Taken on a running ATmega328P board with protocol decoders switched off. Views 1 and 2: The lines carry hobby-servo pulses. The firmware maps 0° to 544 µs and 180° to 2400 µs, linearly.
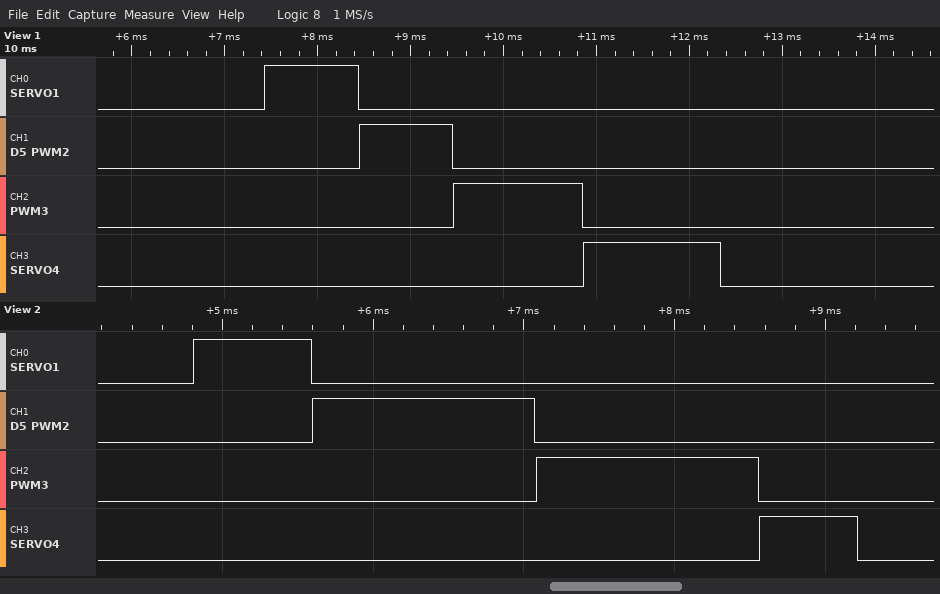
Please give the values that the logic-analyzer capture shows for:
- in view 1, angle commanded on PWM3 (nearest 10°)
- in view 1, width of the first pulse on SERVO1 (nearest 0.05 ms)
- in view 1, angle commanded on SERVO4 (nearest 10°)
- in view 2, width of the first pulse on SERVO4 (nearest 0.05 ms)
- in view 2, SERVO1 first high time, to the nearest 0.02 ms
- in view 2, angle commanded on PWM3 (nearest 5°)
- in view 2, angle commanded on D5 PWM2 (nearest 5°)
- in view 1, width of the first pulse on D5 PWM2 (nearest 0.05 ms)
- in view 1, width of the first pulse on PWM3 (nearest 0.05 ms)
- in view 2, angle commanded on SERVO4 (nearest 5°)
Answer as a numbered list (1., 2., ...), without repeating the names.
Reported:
1. 80°
2. 1.00 ms
3. 90°
4. 0.65 ms
5. 0.78 ms
6. 90°
7. 90°
8. 1.00 ms
9. 1.40 ms
10. 10°
